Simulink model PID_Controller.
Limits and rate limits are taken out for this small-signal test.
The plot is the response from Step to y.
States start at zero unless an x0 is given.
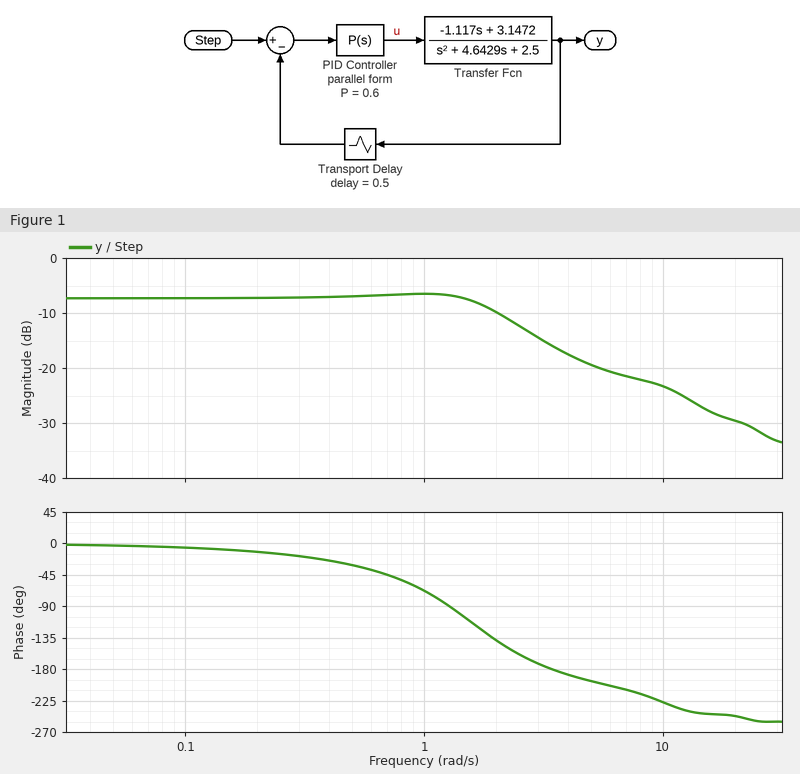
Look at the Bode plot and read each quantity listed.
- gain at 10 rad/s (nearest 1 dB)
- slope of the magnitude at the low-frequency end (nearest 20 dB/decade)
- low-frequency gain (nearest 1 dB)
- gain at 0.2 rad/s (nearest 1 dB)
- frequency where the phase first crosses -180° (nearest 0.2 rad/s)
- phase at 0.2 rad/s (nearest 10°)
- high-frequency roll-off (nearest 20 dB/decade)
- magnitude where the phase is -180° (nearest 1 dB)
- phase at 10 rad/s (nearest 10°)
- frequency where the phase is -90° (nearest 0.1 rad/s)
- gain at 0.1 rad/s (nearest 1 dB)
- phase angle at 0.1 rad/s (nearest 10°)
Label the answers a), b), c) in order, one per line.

a) -23 dB
b) 0 dB/decade
c) -7 dB
d) -7 dB
e) 3.4 rad/s
f) -10°
g) -20 dB/decade
h) -16 dB
i) -230°
j) 1.3 rad/s
k) -7 dB
l) -10°
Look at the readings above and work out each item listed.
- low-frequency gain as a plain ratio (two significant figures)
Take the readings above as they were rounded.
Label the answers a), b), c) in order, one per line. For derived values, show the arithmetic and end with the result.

a) 10^(-7 / 20) = 0.45
